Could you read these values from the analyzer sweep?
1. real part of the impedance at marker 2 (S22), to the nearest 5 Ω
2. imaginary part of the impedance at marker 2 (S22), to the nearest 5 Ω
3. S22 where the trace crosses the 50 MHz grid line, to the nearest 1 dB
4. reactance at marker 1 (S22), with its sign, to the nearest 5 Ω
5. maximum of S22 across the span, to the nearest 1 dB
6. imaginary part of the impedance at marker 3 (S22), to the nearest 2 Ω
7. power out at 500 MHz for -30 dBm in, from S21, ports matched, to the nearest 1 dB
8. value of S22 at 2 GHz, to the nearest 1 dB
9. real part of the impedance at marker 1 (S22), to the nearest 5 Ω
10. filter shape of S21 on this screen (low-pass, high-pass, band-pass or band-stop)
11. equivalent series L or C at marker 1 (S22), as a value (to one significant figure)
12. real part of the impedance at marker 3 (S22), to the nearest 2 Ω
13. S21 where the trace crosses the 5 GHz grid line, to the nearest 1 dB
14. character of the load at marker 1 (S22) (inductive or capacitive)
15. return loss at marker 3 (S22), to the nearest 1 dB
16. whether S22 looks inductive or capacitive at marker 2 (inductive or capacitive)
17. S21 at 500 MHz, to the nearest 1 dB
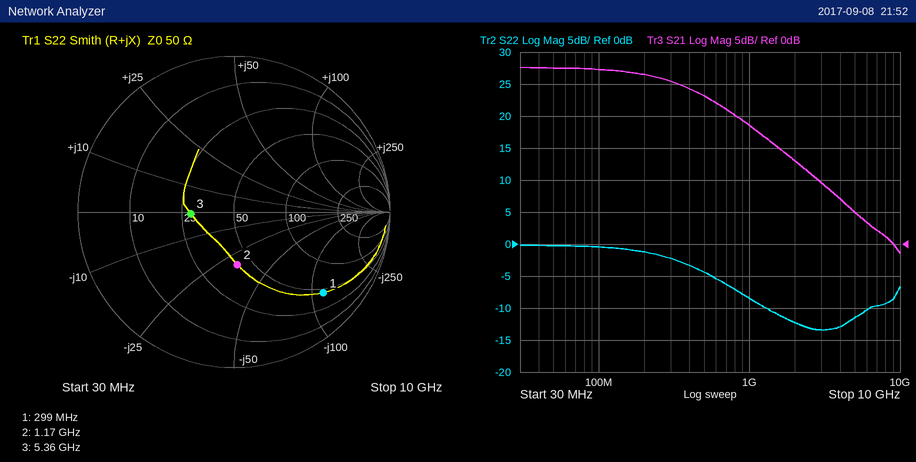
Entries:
40 Ω
-30 Ω
0 dB
-115 Ω
0 dB
0 Ω
-7 dBm
-12 dB
45 Ω
low-pass
5 pF
28 Ω
5 dB
capacitive
11 dB
capacitive
23 dB
